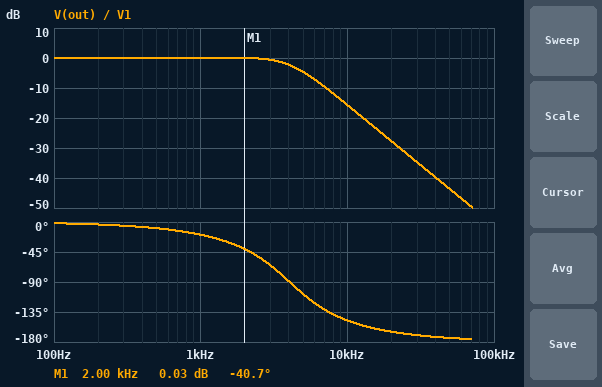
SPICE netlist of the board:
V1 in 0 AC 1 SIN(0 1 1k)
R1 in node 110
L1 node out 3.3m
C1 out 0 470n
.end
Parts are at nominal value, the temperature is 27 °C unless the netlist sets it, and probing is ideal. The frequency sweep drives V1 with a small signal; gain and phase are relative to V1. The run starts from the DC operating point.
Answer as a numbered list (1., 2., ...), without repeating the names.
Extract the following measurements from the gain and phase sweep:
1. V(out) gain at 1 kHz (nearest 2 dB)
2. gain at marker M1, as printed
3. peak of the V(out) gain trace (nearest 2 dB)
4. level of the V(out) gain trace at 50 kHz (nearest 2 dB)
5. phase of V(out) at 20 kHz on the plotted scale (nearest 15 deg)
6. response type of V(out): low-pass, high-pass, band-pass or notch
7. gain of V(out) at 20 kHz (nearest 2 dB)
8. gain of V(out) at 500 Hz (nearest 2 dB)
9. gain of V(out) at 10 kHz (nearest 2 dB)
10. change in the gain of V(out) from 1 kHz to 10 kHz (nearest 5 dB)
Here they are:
1. 0 dB
2. 0.03 dB
3. 0 dB
4. -44 dB
5. -165 deg
6. low-pass
7. -28 dB
8. 0 dB
9. -16 dB
10. -15 dB
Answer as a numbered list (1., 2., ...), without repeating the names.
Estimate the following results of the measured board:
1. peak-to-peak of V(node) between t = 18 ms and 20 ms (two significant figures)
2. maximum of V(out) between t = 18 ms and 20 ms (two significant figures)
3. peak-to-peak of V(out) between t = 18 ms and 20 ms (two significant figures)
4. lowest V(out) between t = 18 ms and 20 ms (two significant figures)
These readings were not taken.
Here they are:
1. 1.9 V
2. 1.0 V
3. 2.0 V
4. -1.0 V
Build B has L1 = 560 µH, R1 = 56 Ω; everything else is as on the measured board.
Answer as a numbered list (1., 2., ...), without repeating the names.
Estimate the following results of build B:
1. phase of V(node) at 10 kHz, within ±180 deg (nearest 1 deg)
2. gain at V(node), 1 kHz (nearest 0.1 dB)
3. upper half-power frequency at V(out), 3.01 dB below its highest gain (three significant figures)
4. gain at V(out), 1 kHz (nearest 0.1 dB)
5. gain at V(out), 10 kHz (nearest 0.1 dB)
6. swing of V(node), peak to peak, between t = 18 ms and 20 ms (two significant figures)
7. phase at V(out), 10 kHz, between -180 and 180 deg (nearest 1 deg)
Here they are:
1. 89 deg
2. -0.1 dB
3. 8.40 kHz
4. 0 dB
5. -4.4 dB
6. 2.0 V
7. -91 deg
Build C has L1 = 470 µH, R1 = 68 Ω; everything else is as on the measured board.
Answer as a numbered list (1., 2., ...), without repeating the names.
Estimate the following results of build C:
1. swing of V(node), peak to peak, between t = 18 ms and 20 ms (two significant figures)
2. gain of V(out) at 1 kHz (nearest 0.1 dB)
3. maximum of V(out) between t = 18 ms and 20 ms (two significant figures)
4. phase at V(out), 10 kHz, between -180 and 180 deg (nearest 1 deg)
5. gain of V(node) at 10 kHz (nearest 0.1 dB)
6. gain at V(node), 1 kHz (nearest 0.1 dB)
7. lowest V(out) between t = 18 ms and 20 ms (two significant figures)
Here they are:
1. 2.0 V
2. -0.1 dB
3. 990 mV
4. -86 deg
5. -23.9 dB
6. -0.2 dB
7. -990 mV
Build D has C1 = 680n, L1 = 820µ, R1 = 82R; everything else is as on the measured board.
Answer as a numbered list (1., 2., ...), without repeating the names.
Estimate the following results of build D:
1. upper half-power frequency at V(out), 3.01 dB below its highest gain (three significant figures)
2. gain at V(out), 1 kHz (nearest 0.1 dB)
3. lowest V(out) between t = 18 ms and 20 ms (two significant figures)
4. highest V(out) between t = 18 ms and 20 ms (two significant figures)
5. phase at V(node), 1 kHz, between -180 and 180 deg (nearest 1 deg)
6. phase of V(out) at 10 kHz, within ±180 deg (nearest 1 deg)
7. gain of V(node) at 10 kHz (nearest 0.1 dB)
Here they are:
1. 3.44 kHz
2. -0.3 dB
3. -960 mV
4. 960 mV
5. -20 deg
6. -109 deg
7. -9.8 dB
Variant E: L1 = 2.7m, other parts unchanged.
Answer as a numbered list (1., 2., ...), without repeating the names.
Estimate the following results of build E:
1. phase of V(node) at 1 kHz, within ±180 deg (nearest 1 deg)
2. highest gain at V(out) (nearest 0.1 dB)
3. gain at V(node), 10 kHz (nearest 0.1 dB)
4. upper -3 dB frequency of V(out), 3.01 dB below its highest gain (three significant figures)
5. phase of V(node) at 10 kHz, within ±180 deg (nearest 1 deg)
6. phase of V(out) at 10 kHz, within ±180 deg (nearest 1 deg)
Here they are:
1. -19 deg
2. 0 dB
3. -2.2 dB
4. 4.35 kHz
5. 39 deg
6. -141 deg
